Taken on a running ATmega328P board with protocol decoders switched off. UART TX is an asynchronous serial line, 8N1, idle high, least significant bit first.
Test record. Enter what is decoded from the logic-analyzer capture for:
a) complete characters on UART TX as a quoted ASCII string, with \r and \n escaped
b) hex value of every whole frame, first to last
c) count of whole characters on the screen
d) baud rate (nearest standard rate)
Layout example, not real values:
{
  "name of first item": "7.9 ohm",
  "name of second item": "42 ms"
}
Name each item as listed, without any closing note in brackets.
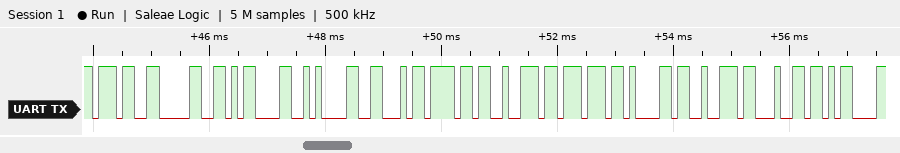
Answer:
{
  "complete characters on UART TX as a quoted ASCII string, with \\r and \\n escaped": "\"70\\r\\nForward\\r\"",
  "hex value of every whole frame, first to last": "0x37 0x30 0x0D 0x0A 0x46 0x6F 0x72 0x77 0x61 0x72 0x64 0x0D",
  "count of whole characters on the screen": "12",
  "baud rate": "9600 baud"
}
